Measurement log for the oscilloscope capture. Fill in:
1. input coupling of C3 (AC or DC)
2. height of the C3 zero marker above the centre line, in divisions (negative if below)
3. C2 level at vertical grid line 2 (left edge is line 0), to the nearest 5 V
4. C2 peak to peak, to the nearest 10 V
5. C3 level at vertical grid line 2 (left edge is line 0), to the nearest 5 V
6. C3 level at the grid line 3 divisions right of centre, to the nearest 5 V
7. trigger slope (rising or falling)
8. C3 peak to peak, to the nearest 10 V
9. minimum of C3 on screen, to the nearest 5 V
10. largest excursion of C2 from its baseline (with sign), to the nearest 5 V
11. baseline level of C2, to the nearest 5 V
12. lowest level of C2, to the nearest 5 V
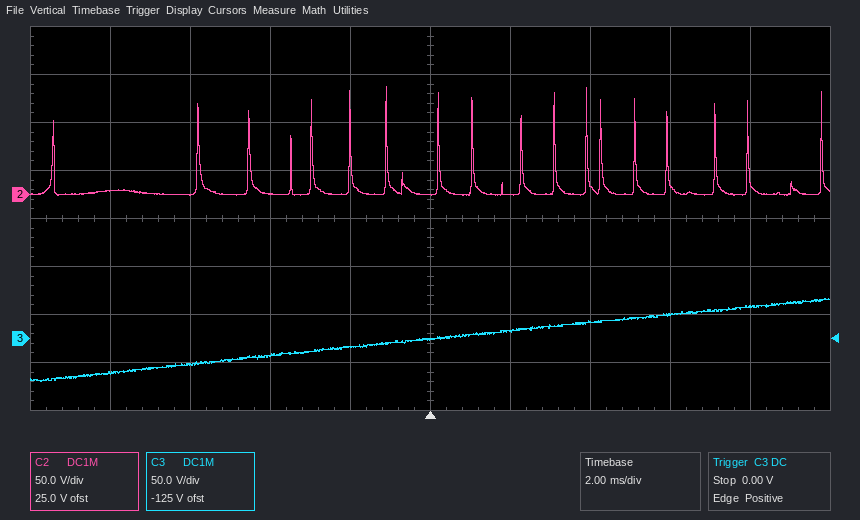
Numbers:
DC
-2.5 div
0 V
110 V
-25 V
25 V
rising
90 V
-45 V
+110 V
0 V
0 V
